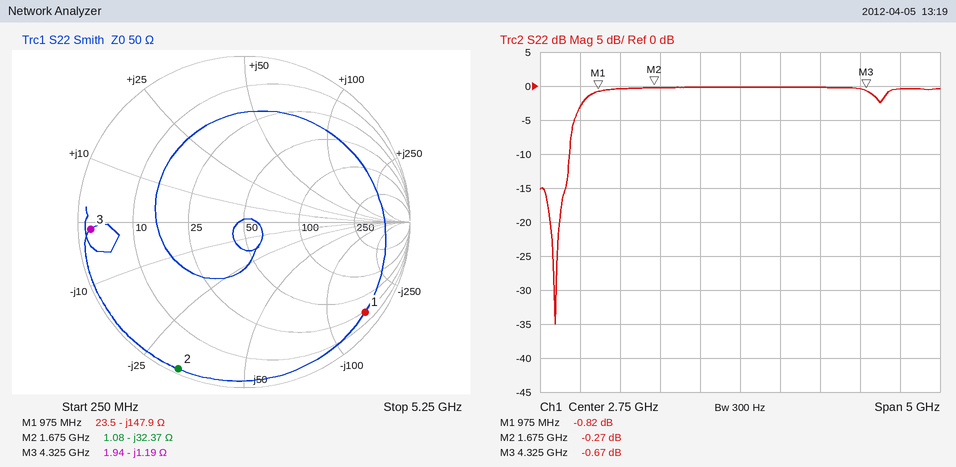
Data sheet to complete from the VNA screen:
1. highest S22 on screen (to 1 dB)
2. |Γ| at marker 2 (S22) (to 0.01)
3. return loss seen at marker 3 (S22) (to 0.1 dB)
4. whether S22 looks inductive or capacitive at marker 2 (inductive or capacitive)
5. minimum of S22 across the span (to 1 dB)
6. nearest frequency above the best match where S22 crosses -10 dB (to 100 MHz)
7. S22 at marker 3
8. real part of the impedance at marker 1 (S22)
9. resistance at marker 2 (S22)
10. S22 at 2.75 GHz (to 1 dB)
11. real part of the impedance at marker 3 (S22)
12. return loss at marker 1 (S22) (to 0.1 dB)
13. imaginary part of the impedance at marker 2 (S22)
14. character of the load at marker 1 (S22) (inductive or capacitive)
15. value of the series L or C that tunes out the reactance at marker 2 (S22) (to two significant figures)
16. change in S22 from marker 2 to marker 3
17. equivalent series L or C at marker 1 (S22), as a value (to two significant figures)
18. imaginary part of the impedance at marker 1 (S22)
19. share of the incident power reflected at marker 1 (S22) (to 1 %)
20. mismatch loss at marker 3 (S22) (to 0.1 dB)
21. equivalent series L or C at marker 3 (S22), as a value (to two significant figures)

0 dB
0.97
0.7 dB
capacitive
-35 dB
600 MHz
-0.67 dB
23.5 Ω
1.08 Ω
0 dB
1.94 Ω
0.8 dB
-32.37 Ω
capacitive
3.1 nH
-0.40 dB
1.1 pF
-147.9 Ω
83 %
8.4 dB
31 pF
